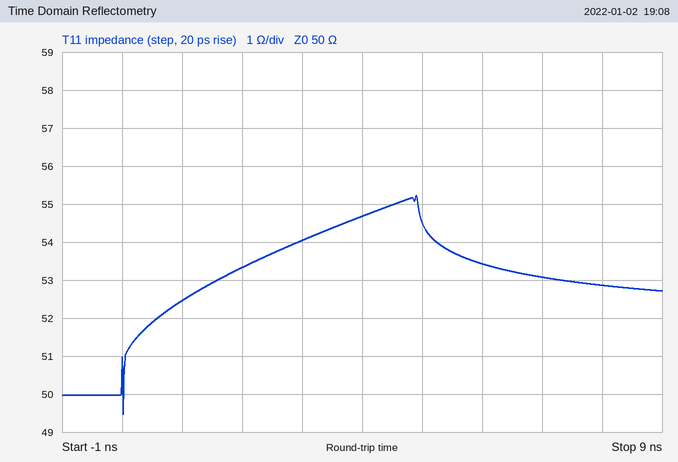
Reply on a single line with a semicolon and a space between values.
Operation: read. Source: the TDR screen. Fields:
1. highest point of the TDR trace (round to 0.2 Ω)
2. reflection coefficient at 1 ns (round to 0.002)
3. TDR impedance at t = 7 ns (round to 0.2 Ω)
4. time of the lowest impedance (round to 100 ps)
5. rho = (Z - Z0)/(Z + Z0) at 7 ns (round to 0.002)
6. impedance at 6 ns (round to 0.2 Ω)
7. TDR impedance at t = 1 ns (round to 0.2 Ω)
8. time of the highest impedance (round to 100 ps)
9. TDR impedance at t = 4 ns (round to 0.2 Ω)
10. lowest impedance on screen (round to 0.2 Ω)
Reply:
55.2 Ω; +0.024; 53.0 Ω; 0.0 ns; +0.030; 53.4 Ω; 52.4 Ω; 4.9 ns; 54.6 Ω; 49.4 Ω
